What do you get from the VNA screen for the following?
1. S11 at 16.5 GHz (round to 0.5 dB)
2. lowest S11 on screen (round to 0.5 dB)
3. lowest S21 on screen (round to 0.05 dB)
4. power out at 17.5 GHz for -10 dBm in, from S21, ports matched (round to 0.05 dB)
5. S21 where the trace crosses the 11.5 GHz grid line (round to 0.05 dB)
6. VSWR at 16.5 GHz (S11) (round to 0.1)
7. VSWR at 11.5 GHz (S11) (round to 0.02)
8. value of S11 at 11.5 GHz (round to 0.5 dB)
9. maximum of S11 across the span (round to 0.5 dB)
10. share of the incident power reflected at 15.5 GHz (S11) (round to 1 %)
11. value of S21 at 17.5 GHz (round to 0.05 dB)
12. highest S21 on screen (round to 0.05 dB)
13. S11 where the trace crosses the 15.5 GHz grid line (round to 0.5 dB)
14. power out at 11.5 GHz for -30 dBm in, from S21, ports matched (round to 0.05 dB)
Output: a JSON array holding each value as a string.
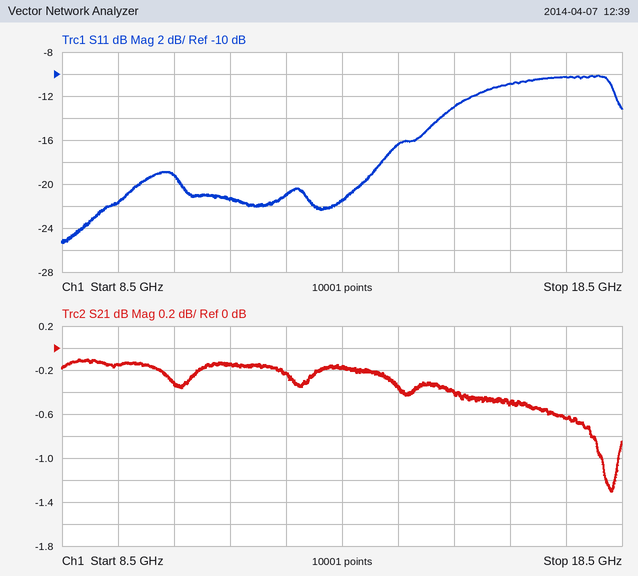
["-11.0 dB", "-25.5 dB", "-1.30 dB", "-10.65 dBm", "-0.15 dB", "1.8", "1.18", "-21.5 dB", "-10.0 dB", "5 %", "-0.65 dB", "-0.10 dB", "-13.0 dB", "-30.15 dBm"]
